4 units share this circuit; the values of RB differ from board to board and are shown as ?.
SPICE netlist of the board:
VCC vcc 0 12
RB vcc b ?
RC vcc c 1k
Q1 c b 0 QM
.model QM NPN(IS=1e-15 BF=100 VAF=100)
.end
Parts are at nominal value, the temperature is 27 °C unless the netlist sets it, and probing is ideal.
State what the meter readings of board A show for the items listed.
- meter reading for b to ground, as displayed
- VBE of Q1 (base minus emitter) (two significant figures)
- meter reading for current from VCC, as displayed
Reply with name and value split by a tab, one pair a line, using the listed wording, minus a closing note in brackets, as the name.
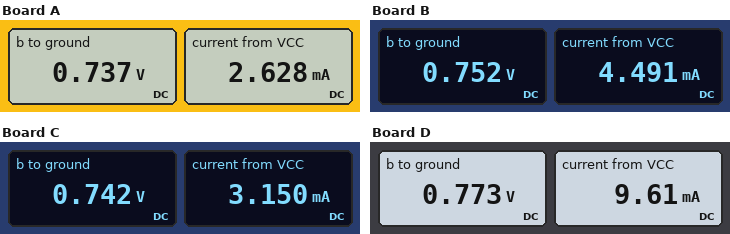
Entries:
meter reading for b to ground, as displayed	0.737 V
VBE of Q1 (base minus emitter)	740 mV
meter reading for current from VCC, as displayed	2.628 mA
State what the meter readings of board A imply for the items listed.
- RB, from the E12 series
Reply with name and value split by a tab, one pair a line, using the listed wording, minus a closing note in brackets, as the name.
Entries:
RB, from the E12 series	470 kΩ
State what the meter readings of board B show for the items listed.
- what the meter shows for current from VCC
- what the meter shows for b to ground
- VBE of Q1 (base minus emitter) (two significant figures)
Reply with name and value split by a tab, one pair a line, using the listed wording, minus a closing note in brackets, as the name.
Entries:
what the meter shows for current from VCC	4.491 mA
what the meter shows for b to ground	0.752 V
VBE of Q1 (base minus emitter)	750 mV
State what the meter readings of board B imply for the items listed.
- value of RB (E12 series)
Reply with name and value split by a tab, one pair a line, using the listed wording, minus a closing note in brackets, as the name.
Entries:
value of RB	270 kΩ
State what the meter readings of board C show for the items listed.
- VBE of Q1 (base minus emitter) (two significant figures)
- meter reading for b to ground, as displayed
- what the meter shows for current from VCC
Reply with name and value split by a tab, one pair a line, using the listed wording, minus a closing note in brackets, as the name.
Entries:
VBE of Q1 (base minus emitter)	740 mV
meter reading for b to ground, as displayed	0.742 V
what the meter shows for current from VCC	3.150 mA
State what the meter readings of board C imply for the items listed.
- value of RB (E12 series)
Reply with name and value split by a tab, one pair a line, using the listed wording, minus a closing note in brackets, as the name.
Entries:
value of RB	390 kΩ
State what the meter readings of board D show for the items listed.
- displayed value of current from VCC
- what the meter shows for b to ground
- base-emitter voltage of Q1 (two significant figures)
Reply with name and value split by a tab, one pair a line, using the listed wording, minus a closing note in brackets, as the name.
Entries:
displayed value of current from VCC	9.61 mA
what the meter shows for b to ground	0.773 V
base-emitter voltage of Q1	770 mV
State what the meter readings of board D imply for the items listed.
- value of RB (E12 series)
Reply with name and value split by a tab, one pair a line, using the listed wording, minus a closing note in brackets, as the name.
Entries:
value of RB	120 kΩ
